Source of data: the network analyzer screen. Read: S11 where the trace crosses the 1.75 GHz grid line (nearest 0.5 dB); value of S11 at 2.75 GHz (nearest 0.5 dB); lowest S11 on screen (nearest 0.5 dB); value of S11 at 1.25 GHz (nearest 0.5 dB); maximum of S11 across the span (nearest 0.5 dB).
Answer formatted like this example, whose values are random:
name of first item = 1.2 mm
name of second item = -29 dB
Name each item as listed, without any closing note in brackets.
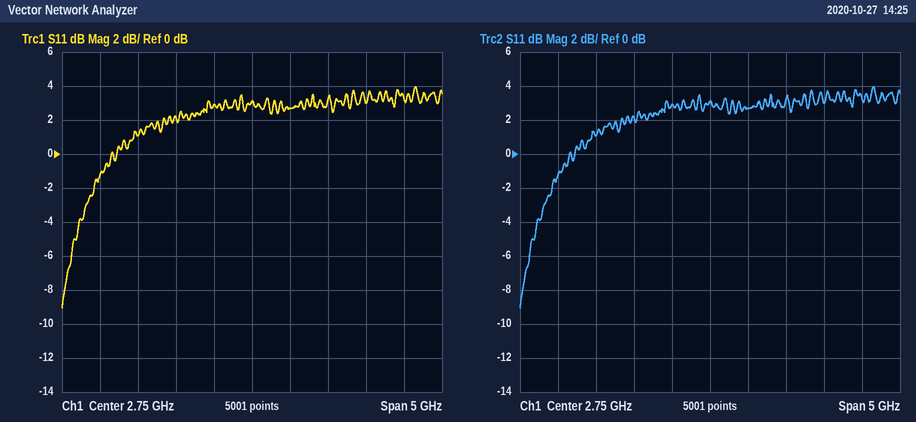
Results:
S11 where the trace crosses the 1.75 GHz grid line = 2.0 dB
value of S11 at 2.75 GHz = 3.0 dB
lowest S11 on screen = -9.0 dB
value of S11 at 1.25 GHz = 1.0 dB
maximum of S11 across the span = 4.0 dB
